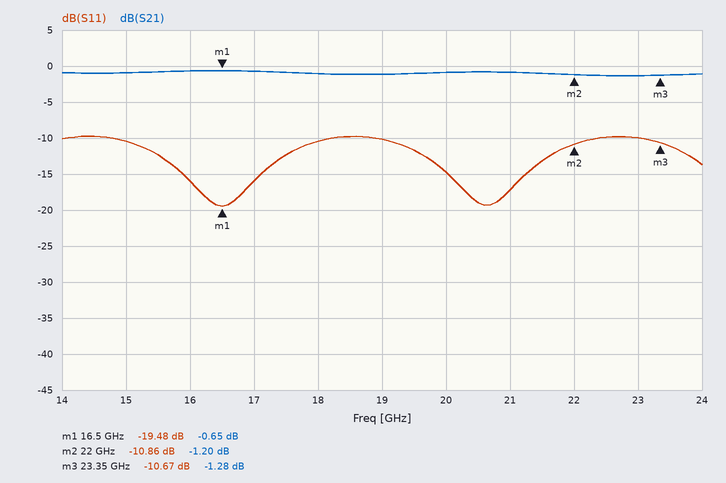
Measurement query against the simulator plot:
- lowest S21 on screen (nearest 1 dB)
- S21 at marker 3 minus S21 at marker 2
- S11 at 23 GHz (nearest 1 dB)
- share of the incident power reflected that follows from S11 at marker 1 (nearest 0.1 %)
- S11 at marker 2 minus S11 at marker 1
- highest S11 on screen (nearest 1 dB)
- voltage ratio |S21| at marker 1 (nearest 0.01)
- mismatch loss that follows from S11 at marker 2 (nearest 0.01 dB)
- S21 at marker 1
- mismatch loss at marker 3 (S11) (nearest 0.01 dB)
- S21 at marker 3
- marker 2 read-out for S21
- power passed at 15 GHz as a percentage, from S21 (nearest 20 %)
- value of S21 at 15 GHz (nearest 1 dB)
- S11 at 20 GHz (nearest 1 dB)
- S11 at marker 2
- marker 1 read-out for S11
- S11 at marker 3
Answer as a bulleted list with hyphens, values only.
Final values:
- -1 dB
- -0.08 dB
- -10 dB
- 1.1 %
- 8.62 dB
- -10 dB
- 0.93
- 0.37 dB
- -0.65 dB
- 0.39 dB
- -1.28 dB
- -1.20 dB
- 80 %
- -1 dB
- -15 dB
- -10.86 dB
- -19.48 dB
- -10.67 dB
